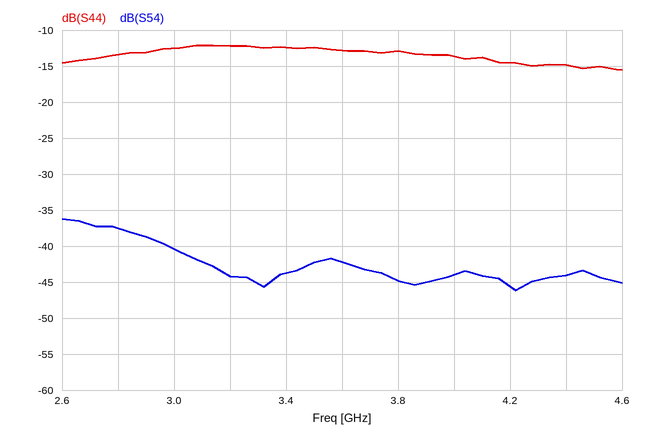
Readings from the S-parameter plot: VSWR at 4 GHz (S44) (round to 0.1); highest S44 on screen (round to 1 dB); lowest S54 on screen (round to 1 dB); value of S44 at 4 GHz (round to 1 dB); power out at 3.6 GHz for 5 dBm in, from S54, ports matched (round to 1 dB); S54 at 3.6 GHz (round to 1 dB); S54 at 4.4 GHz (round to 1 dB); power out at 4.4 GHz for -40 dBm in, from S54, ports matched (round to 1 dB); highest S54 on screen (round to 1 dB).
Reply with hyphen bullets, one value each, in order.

- 1.5
- -12 dB
- -46 dB
- -14 dB
- -37 dBm
- -42 dB
- -44 dB
- -84 dBm
- -36 dB
